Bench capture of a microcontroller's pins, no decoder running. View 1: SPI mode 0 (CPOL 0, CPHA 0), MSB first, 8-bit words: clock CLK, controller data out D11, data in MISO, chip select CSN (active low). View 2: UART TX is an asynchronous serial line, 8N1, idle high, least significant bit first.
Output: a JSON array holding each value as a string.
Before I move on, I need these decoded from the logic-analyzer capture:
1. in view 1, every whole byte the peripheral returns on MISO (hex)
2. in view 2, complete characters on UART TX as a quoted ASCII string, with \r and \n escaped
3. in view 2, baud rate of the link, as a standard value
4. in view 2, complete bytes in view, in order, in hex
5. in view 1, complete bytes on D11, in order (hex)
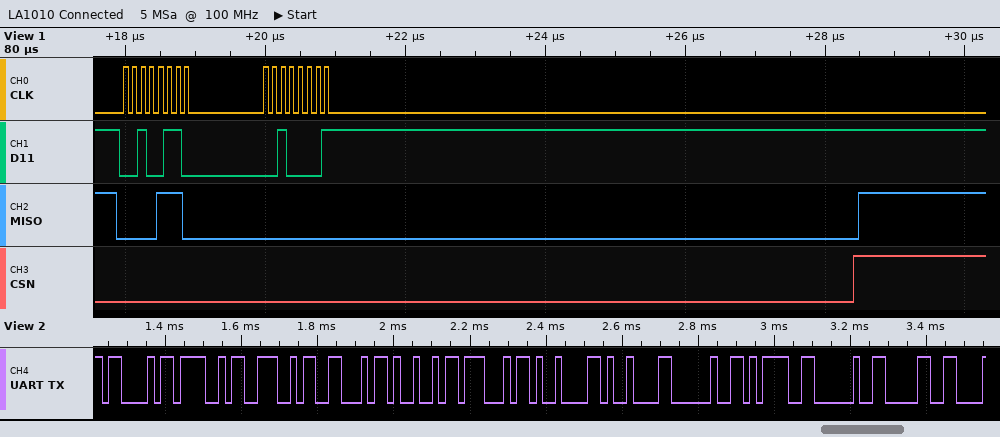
["0E 00", "\"CONFIG\\t\\t = 0\"", "57600 baud", "43 4F 4E 46 49 47 09 09 20 3D 20 30", "26 21"]
